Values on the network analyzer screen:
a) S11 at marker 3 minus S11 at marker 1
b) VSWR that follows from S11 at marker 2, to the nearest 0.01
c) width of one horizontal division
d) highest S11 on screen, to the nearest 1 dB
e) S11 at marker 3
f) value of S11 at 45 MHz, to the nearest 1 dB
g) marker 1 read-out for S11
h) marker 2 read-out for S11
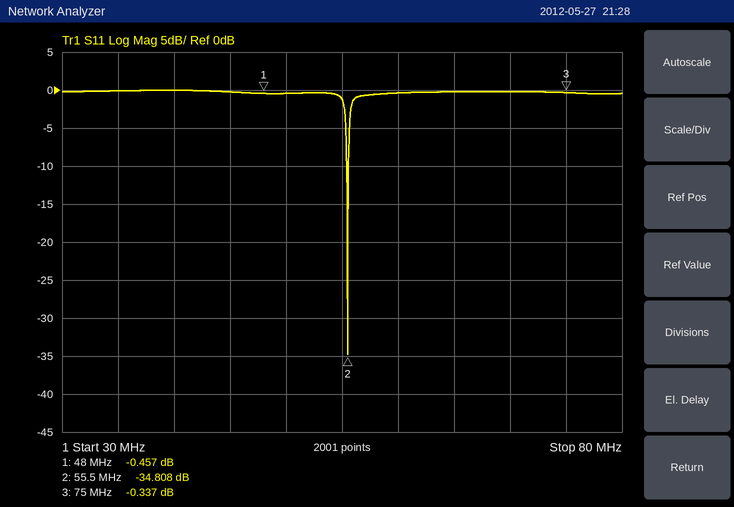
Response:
0.120 dB
1.04
5 MHz
0 dB
-0.337 dB
0 dB
-0.457 dB
-34.808 dB
